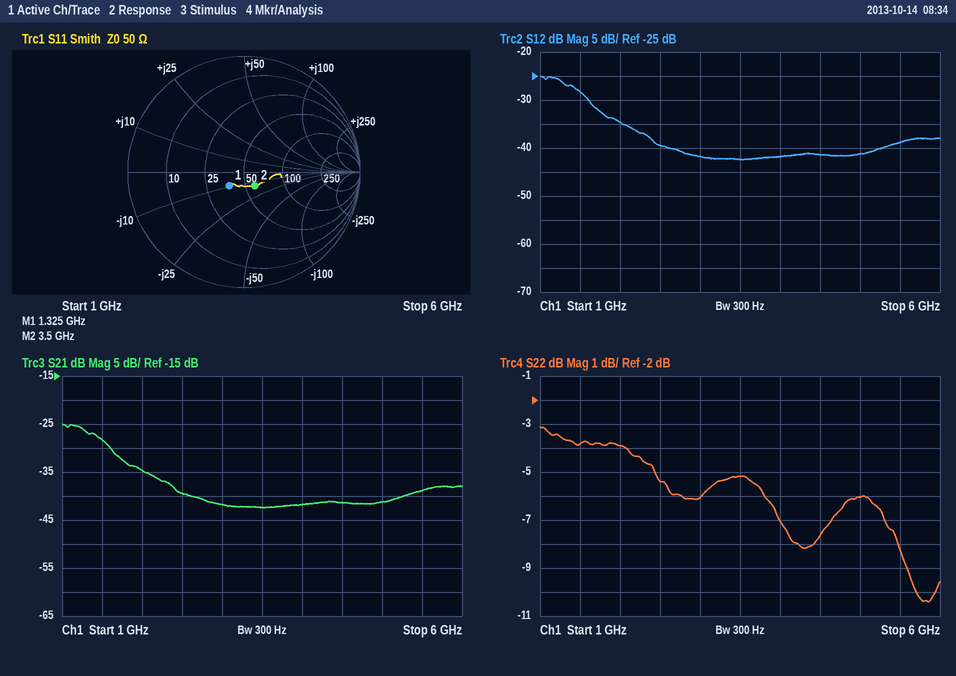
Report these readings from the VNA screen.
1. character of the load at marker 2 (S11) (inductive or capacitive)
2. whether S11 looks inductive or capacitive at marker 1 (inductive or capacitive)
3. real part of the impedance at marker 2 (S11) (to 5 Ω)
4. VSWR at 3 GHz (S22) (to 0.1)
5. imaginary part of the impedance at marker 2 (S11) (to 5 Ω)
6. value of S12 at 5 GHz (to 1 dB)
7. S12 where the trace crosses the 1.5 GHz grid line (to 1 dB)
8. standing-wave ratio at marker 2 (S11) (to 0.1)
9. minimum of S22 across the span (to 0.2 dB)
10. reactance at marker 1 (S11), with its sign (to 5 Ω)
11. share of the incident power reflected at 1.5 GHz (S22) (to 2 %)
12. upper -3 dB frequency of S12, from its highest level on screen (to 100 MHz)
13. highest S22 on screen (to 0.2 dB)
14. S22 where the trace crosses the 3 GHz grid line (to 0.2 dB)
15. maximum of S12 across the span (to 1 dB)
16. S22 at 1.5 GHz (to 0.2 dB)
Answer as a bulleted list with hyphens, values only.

- capacitive
- capacitive
- 60 Ω
- 3.0
- -15 Ω
- -41 dB
- -28 dB
- 1.4
- -10.4 dB
- -10 Ω
- 42 %
- 1.5 GHz
- -3.2 dB
- -6.0 dB
- -25 dB
- -3.8 dB
